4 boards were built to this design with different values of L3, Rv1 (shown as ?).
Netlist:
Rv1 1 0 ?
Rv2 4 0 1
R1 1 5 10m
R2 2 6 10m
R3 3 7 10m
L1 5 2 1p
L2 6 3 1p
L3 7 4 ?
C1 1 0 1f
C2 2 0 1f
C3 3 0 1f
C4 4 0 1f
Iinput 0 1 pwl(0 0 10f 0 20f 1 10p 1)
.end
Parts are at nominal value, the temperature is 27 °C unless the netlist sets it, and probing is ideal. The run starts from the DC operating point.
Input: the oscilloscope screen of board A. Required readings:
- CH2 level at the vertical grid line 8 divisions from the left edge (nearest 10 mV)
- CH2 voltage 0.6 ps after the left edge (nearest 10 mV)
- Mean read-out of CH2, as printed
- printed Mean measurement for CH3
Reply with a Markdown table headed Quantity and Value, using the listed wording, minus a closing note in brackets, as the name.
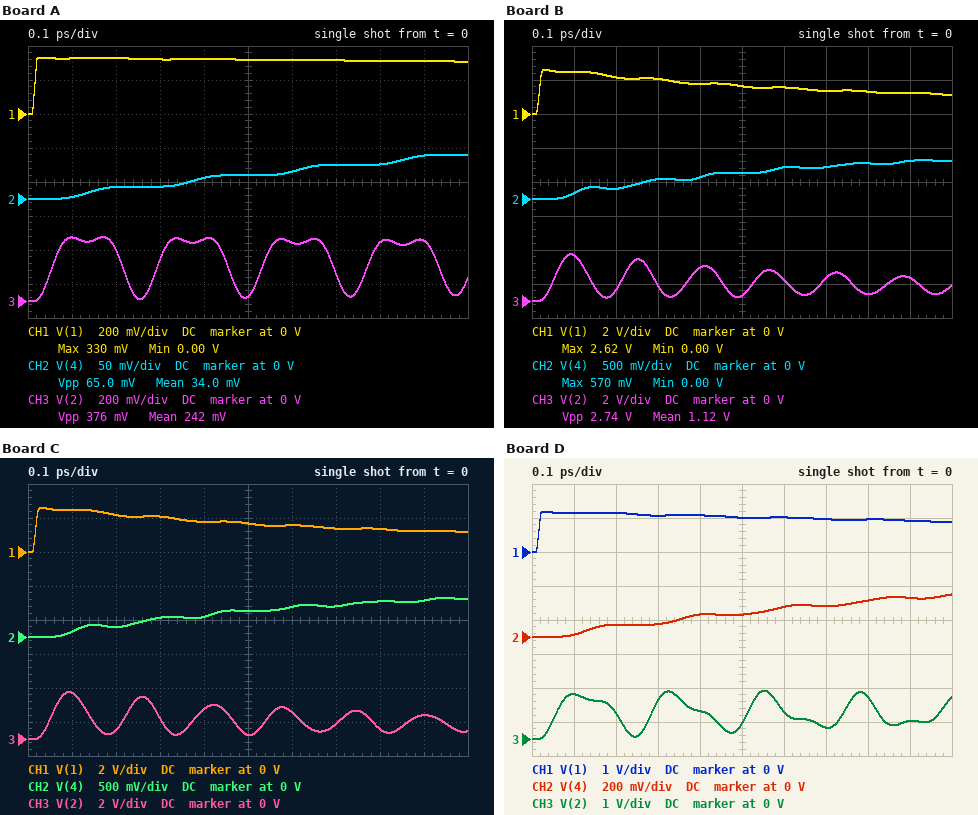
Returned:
| Quantity | Value |
|---|---|
| CH2 level at the vertical grid line 8 divisions from the left edge | 50 mV |
| CH2 voltage 0.6 ps after the left edge | 40 mV |
| Mean read-out of CH2, as printed | 34.0 mV |
| printed Mean measurement for CH3 | 242 mV |
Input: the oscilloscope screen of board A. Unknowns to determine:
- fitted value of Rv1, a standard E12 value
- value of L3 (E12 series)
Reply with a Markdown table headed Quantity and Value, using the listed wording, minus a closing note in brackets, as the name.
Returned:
| Quantity | Value |
|---|---|
| fitted value of Rv1, a standard E12 value | 0.33 Ω |
| value of L3 | 2.2 pH |
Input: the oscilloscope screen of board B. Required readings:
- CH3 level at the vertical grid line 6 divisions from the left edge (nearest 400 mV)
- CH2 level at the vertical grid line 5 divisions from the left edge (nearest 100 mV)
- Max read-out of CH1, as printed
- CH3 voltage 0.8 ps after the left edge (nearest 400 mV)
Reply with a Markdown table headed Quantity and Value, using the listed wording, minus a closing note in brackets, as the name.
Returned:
| Quantity | Value |
|---|---|
| CH3 level at the vertical grid line 6 divisions from the left edge | 1.2 V |
| CH2 level at the vertical grid line 5 divisions from the left edge | 400 mV |
| Max read-out of CH1, as printed | 2.62 V |
| CH3 voltage 0.8 ps after the left edge | 400 mV |
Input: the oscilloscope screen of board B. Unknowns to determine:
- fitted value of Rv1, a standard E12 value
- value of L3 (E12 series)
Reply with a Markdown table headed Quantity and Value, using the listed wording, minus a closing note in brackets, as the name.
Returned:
| Quantity | Value |
|---|---|
| fitted value of Rv1, a standard E12 value | 2.7 Ω |
| value of L3 | 330 fH |
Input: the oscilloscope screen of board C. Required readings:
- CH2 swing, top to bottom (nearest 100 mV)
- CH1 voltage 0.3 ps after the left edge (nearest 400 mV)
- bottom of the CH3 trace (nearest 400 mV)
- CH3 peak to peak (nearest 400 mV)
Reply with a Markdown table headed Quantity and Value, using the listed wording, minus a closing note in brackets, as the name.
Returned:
| Quantity | Value |
|---|---|
| CH2 swing, top to bottom | 600 mV |
| CH1 voltage 0.3 ps after the left edge | 2.0 V |
| bottom of the CH3 trace | 0 V |
| CH3 peak to peak | 2.8 V |
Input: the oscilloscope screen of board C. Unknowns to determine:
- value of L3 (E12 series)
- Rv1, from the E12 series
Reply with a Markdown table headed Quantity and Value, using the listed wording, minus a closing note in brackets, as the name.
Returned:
| Quantity | Value |
|---|---|
| value of L3 | 390 fH |
| Rv1, from the E12 series | 2.7 Ω |
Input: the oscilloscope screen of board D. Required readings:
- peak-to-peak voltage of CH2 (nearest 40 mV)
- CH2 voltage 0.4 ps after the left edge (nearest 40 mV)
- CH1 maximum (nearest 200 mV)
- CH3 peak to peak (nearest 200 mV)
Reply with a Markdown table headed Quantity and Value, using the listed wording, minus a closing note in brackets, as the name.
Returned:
| Quantity | Value |
|---|---|
| peak-to-peak voltage of CH2 | 240 mV |
| CH2 voltage 0.4 ps after the left edge | 120 mV |
| CH1 maximum | 1.2 V |
| CH3 peak to peak | 1.4 V |
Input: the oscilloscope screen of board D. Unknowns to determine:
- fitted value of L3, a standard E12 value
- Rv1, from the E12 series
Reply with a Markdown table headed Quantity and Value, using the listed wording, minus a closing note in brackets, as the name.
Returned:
| Quantity | Value |
|---|---|
| fitted value of L3, a standard E12 value | 1.5 pH |
| Rv1, from the E12 series | 1.2 Ω |
